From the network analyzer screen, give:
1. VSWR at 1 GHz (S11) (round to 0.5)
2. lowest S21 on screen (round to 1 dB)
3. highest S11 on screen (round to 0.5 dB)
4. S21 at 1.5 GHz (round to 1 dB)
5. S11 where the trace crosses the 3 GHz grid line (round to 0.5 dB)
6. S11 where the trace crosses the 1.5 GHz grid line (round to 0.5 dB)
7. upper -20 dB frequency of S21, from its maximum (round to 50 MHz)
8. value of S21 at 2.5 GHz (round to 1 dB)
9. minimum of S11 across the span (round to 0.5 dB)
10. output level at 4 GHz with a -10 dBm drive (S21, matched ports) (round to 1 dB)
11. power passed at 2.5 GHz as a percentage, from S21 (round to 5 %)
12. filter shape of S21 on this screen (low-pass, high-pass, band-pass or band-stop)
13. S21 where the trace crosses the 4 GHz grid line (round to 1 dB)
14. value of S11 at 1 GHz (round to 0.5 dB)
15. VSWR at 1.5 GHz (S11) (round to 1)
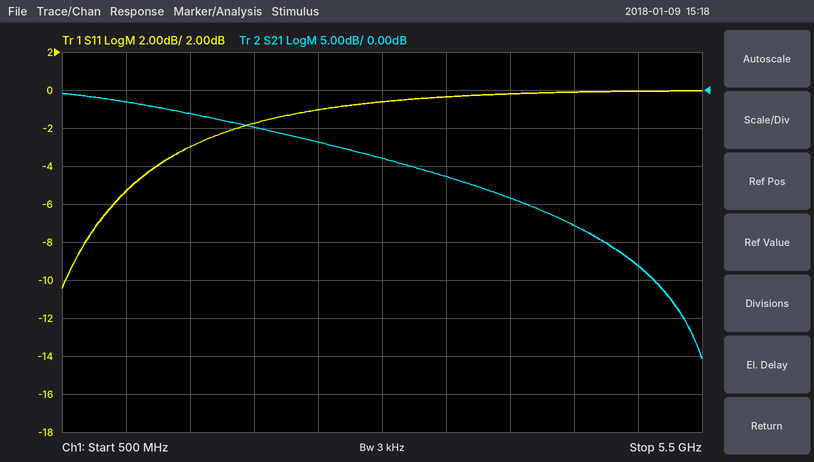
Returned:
3.5
-35 dB
0.0 dB
-3 dB
-0.5 dB
-3.0 dB
4.80 GHz
-7 dB
-10.5 dB
-24 dBm
20 %
low-pass
-14 dB
-5.5 dB
6
